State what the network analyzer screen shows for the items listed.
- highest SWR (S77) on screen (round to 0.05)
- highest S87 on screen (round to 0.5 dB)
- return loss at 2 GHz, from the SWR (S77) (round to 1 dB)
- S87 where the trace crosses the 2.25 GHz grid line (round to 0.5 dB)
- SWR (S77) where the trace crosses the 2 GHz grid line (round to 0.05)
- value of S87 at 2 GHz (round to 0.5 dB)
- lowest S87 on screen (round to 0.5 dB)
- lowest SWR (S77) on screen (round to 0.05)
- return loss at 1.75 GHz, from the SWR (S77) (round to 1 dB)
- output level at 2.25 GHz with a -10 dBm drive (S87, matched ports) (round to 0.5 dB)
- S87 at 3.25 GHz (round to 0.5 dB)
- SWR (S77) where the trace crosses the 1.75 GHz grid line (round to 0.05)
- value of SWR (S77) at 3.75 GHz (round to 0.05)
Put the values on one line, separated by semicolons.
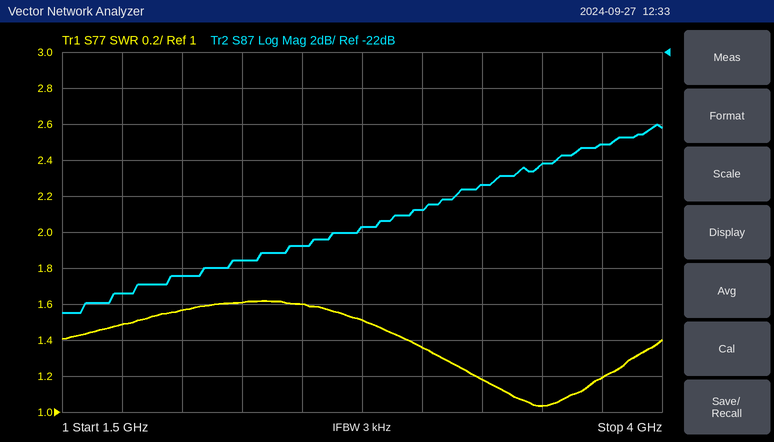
1.60; -26.0 dB; 13 dB; -33.5 dB; 1.55; -34.5 dB; -36.5 dB; 1.05; 14 dB; -43.5 dBm; -29.5 dB; 1.50; 1.20
